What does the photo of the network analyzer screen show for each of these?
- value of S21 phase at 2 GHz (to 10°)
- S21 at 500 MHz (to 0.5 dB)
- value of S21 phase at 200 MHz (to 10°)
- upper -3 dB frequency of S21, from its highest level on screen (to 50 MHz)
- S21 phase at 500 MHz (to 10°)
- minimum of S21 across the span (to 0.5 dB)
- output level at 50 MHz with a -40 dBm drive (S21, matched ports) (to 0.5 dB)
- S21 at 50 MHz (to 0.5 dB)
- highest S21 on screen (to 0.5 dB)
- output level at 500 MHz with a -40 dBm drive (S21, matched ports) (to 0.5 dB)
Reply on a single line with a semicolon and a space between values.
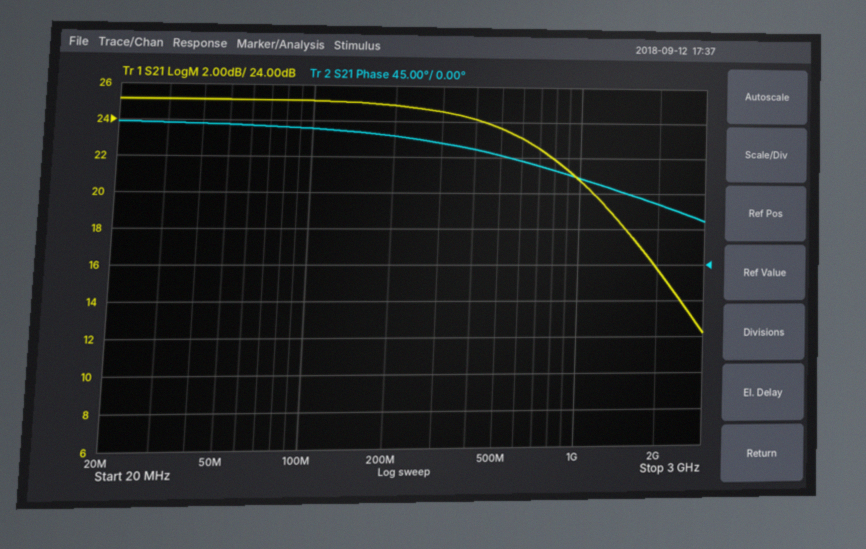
80°; 23.5 dB; 160°; 750 MHz; 140°; 12.0 dB; -15.0 dBm; 25.0 dB; 25.0 dB; -16.5 dBm
